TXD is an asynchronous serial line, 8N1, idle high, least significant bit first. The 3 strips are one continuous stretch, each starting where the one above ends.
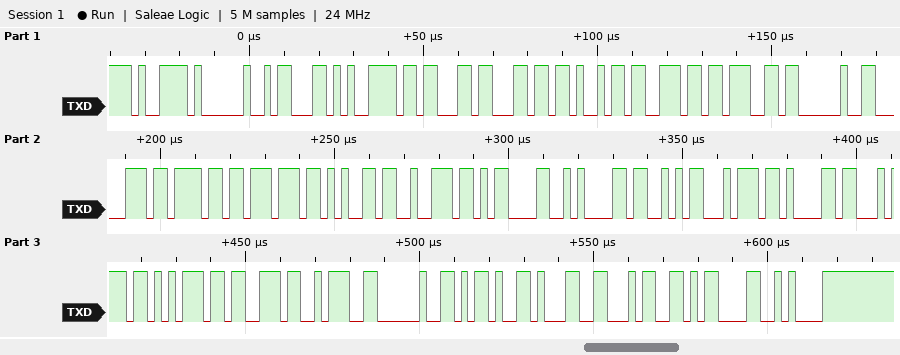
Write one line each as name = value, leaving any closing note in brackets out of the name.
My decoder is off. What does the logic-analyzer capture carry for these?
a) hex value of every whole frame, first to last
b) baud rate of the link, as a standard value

hex value of every whole frame, first to last = 79 20 63 79 63 6C 69 6E 67 20 70 6F 77 65 72 0D 0A 53 74 61 74 75 73 3A 20 2D 31 34 0D 0A
baud rate of the link, as a standard value = 500000 baud
